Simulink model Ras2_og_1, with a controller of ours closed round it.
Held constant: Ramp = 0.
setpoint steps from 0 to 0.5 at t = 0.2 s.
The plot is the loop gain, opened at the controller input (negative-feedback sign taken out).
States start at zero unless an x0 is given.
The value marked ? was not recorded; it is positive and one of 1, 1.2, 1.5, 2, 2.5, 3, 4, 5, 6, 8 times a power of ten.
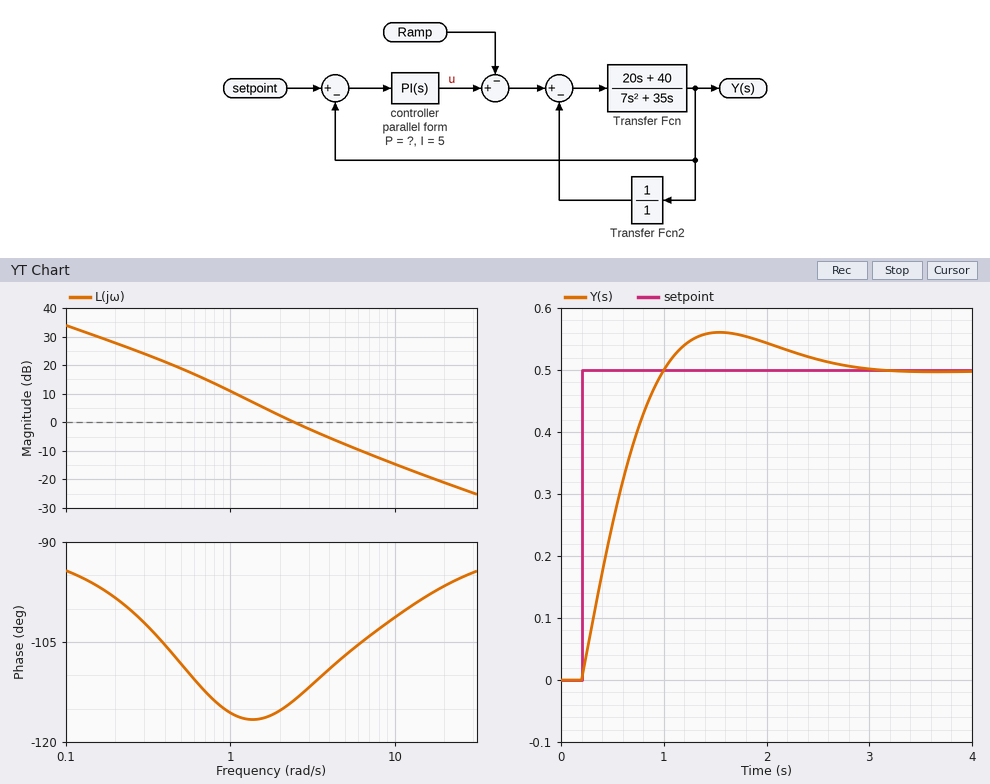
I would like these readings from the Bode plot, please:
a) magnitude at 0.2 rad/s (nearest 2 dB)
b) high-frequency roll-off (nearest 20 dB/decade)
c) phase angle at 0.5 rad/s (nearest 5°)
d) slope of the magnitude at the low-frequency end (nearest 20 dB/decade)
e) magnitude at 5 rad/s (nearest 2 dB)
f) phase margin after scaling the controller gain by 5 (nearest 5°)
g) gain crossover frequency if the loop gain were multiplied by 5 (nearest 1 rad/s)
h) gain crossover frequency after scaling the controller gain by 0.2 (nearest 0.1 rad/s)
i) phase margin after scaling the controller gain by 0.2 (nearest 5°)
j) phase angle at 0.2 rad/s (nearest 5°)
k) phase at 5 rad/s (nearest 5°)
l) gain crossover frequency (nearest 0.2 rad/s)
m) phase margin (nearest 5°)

28 dB
-20 dB/decade
-110°
-20 dB/decade
-8 dB
80°
9 rad/s
0.8 rad/s
65°
-100°
-105°
2.4 rad/s
65°
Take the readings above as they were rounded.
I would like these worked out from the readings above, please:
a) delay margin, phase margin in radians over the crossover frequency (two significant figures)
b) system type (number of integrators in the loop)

0.47 s
1
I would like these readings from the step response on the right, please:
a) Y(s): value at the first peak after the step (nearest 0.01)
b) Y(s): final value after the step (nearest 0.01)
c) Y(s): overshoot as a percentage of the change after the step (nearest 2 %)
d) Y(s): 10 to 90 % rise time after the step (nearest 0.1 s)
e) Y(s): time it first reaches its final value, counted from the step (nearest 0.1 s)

0.56
0.50
12 %
0.6 s
0.8 s
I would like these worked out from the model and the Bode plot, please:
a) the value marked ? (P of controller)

0.6
